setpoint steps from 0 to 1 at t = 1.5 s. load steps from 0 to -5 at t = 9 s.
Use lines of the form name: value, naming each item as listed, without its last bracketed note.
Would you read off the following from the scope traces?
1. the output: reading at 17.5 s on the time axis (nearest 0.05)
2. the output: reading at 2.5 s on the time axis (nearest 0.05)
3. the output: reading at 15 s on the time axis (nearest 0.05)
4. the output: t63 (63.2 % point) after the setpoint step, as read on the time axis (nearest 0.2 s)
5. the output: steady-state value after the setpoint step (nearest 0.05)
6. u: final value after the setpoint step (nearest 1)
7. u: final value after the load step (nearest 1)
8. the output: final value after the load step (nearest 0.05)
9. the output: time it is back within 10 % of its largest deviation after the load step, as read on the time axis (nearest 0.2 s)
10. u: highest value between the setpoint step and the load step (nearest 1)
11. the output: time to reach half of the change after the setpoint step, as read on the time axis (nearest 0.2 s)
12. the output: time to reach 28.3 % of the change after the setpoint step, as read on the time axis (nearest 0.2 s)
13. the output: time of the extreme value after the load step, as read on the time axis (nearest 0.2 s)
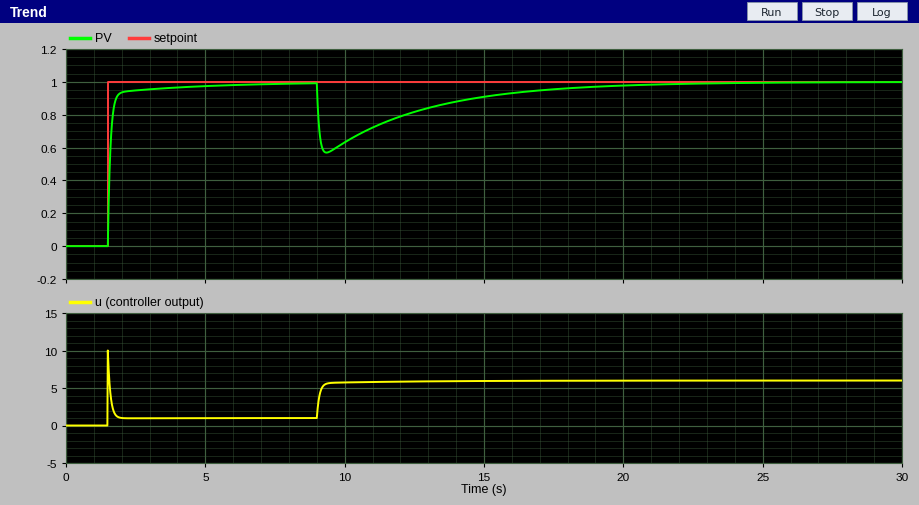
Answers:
the output: reading at 17.5 s on the time axis: 0.95
the output: reading at 2.5 s on the time axis: 0.95
the output: reading at 15 s on the time axis: 0.90
the output: t63 (63.2 % point) after the setpoint step, as read on the time axis: 1.6 s
the output: steady-state value after the setpoint step: 1.00
u: final value after the setpoint step: 1
u: final value after the load step: 6
the output: final value after the load step: 1.00
the output: time it is back within 10 % of its largest deviation after the load step, as read on the time axis: 17.8 s
u: highest value between the setpoint step and the load step: 10
the output: time to reach half of the change after the setpoint step, as read on the time axis: 1.6 s
the output: time to reach 28.3 % of the change after the setpoint step, as read on the time axis: 1.6 s
the output: time of the extreme value after the load step, as read on the time axis: 9.4 s
